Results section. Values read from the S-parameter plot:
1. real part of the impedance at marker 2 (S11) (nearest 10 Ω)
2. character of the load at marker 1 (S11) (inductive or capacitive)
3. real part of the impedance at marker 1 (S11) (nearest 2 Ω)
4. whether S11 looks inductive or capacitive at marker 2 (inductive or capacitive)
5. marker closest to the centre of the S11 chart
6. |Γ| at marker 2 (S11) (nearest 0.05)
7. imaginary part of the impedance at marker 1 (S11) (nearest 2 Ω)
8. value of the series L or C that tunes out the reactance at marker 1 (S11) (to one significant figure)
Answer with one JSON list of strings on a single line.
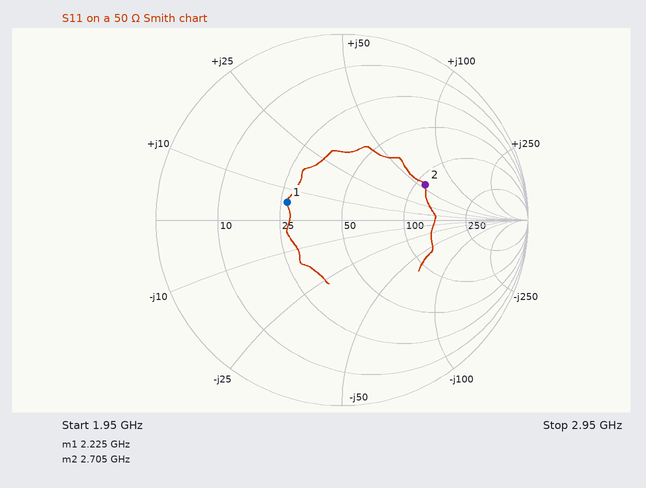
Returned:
["110 Ω", "inductive", "26 Ω", "inductive", "marker 1", "0.50", "+6 Ω", "10 pF"]
